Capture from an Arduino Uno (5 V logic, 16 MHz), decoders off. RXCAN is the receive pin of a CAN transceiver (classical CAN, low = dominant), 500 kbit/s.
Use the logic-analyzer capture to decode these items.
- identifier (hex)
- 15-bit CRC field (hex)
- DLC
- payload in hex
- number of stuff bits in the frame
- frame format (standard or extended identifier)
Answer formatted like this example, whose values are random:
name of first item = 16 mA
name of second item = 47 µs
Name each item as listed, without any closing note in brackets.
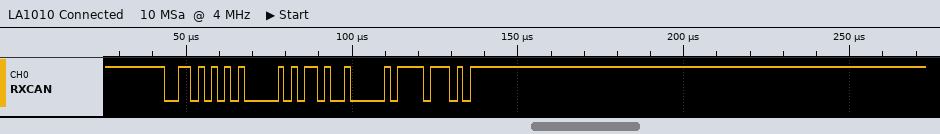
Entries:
identifier = 0x355
15-bit CRC field = 0x01EE
DLC = 1
payload in hex = 69
number of stuff bits in the frame = 2
frame format = standard
